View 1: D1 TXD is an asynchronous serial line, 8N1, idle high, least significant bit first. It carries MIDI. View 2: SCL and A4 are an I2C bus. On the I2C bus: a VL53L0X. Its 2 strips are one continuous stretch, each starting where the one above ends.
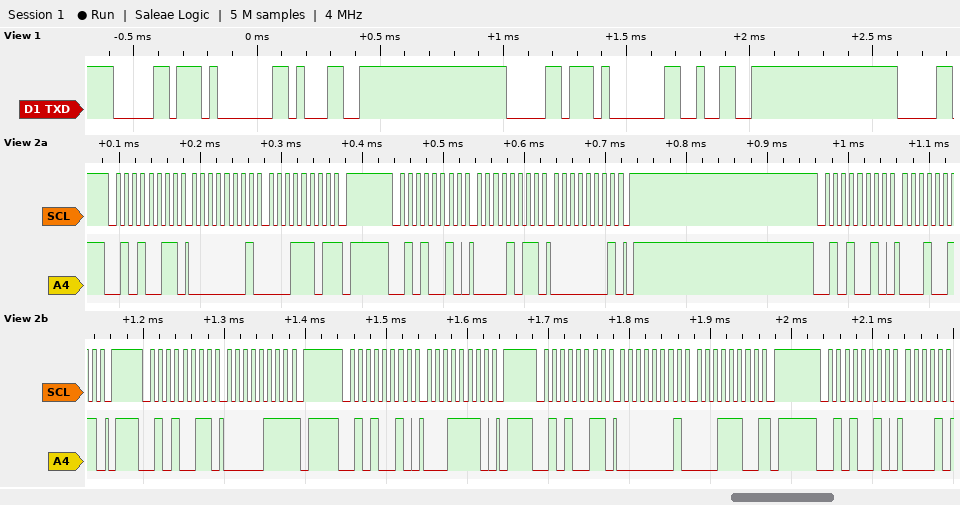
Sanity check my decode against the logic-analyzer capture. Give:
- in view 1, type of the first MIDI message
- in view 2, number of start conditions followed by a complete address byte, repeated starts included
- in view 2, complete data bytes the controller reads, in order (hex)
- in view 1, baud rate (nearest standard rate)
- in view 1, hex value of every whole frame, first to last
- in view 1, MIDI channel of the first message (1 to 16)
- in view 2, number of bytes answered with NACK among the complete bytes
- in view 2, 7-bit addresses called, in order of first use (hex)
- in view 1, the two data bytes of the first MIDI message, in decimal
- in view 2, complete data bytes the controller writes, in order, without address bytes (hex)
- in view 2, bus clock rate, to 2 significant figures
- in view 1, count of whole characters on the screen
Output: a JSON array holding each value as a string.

["Control Change", "7", "01 1D 07 01 1C", "31250 baud", "B0 01 31 B0 01 32", "1", "3", "0x29", "1, 49", "0B 01 13 1E", "100 kHz", "6"]
